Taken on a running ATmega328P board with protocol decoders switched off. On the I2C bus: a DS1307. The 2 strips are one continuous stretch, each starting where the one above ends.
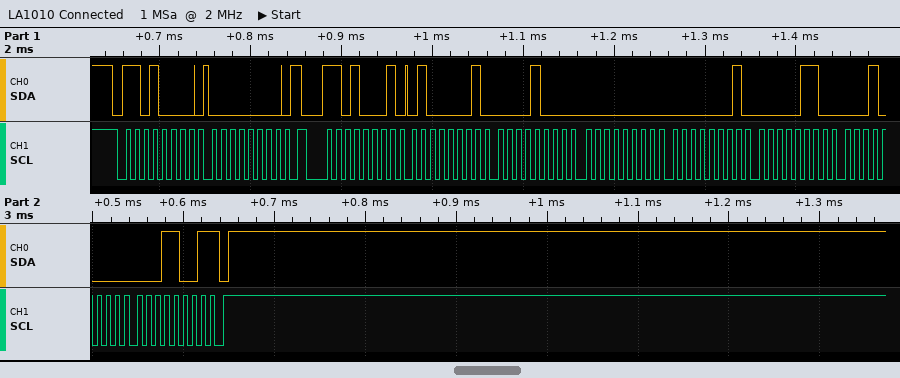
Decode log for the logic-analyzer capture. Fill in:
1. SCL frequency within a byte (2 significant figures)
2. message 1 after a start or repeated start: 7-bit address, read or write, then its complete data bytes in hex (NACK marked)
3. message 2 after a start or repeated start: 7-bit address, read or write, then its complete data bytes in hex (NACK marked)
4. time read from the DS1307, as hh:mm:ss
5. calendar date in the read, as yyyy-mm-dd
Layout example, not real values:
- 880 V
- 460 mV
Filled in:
- 100 kHz
- 0x68 write: 00
- 0x68 read: 41 08 00 01 06 10 19 NACK
- 00:08:41
- 2019-10-06
